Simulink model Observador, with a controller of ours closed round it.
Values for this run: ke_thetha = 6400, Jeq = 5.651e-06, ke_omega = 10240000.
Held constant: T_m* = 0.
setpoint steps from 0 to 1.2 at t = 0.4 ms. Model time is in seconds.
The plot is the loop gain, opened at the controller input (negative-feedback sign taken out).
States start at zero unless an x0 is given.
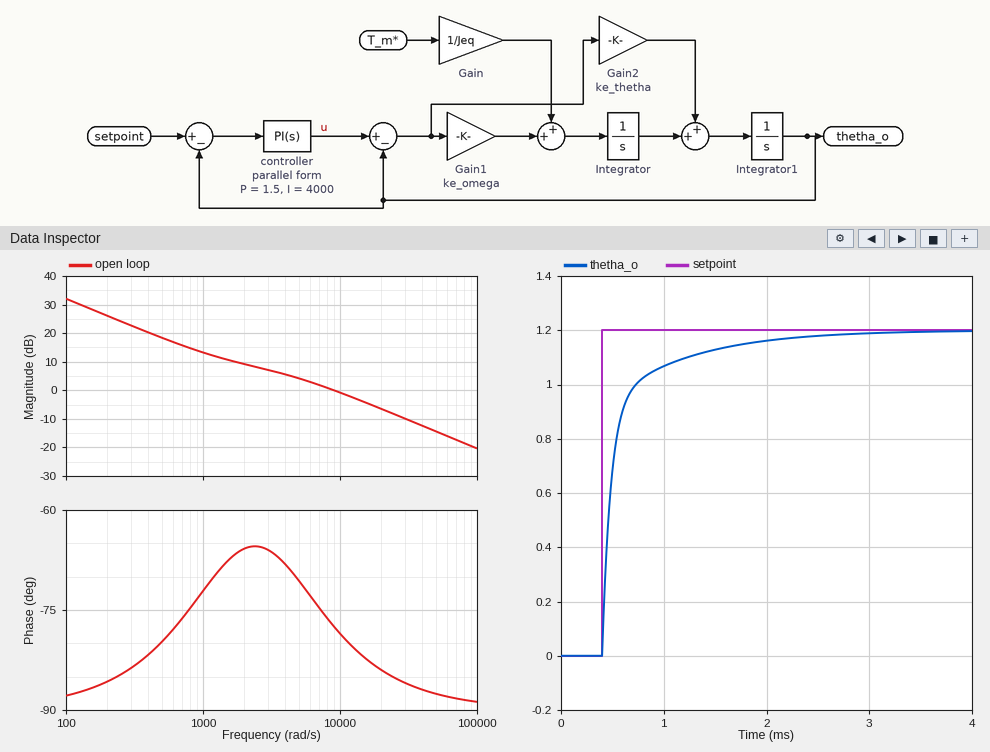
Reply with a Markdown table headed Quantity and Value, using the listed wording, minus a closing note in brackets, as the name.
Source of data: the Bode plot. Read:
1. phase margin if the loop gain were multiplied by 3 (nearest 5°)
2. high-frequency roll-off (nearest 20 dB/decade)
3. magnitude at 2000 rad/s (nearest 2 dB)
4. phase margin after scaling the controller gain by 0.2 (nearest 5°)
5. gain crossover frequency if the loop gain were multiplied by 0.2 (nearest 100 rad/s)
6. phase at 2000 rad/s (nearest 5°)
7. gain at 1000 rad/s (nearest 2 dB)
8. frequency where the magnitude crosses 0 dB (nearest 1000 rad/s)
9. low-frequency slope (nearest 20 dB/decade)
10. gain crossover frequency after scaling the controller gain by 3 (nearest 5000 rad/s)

| Quantity | Value |
|---|---|
| phase margin if the loop gain were multiplied by 3 | 95° |
| high-frequency roll-off | -20 dB/decade |
| magnitude at 2000 rad/s | 10 dB |
| phase margin after scaling the controller gain by 0.2 | 105° |
| gain crossover frequency if the loop gain were multiplied by 0.2 | 900 rad/s |
| phase at 2000 rad/s | -65° |
| gain at 1000 rad/s | 14 dB |
| frequency where the magnitude crosses 0 dB | 9000 rad/s |
| low-frequency slope | -20 dB/decade |
| gain crossover frequency after scaling the controller gain by 3 | 30000 rad/s |
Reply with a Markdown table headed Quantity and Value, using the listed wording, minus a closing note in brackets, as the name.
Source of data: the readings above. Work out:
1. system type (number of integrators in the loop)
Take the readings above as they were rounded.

| Quantity | Value |
|---|---|
| system type | 1 |
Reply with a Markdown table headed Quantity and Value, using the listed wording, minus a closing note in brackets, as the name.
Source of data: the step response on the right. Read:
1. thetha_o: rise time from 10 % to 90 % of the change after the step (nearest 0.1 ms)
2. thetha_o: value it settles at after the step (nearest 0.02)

| Quantity | Value |
|---|---|
| thetha_o: rise time from 10 % to 90 % of the change after the step | 0.7 ms |
| thetha_o: value it settles at after the step | 1.20 |
